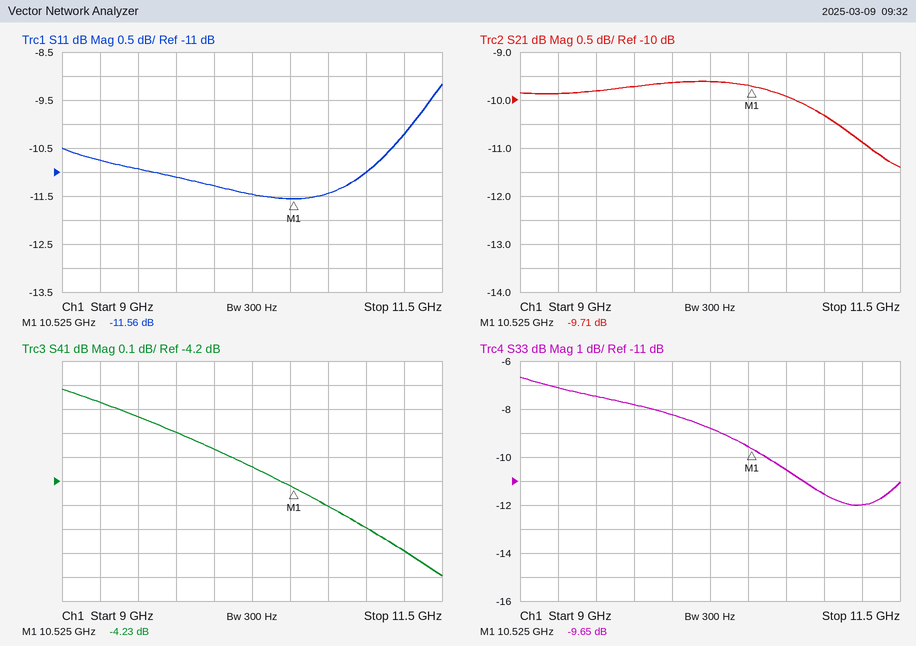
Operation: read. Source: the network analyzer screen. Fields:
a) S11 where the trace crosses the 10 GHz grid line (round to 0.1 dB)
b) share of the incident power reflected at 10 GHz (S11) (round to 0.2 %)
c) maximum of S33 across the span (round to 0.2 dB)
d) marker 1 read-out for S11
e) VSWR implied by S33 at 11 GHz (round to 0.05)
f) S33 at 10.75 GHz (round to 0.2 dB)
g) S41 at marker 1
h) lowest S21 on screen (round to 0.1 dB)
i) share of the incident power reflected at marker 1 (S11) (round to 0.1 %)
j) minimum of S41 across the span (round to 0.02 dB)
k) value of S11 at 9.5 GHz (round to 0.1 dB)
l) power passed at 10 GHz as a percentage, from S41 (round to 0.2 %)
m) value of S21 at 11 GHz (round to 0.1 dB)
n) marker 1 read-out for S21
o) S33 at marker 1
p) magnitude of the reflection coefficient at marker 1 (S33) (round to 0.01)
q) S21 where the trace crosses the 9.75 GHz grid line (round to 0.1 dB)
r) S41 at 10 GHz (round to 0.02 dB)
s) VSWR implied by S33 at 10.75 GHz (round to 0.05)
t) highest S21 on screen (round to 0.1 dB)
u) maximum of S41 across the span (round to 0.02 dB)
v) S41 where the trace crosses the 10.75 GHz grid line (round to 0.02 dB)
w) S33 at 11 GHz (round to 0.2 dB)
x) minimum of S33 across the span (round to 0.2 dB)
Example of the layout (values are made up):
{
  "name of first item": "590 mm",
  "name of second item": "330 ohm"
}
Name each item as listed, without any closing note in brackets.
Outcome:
{
  "S11 where the trace crosses the 10 GHz grid line": "-11.3 dB",
  "share of the incident power reflected at 10 GHz (S11)": "7.4 %",
  "maximum of S33 across the span": "-6.6 dB",
  "marker 1 read-out for S11": "-11.56 dB",
  "VSWR implied by S33 at 11 GHz": "1.70",
  "S33 at 10.75 GHz": "-10.6 dB",
  "S41 at marker 1": "-4.23 dB",
  "lowest S21 on screen": "-11.4 dB",
  "share of the incident power reflected at marker 1 (S11)": "7.0 %",
  "minimum of S41 across the span": "-4.60 dB",
  "value of S11 at 9.5 GHz": "-10.9 dB",
  "power passed at 10 GHz as a percentage, from S41": "39.2 %",
  "value of S21 at 11 GHz": "-10.3 dB",
  "marker 1 read-out for S21": "-9.71 dB",
  "S33 at marker 1": "-9.65 dB",
  "magnitude of the reflection coefficient at marker 1 (S33)": "0.33",
  "S21 where the trace crosses the 9.75 GHz grid line": "-9.7 dB",
  "S41 at 10 GHz": "-4.06 dB",
  "VSWR implied by S33 at 10.75 GHz": "1.85",
  "highest S21 on screen": "-9.6 dB",
  "maximum of S41 across the span": "-3.82 dB",
  "S41 where the trace crosses the 10.75 GHz grid line": "-4.30 dB",
  "S33 at 11 GHz": "-11.6 dB",
  "minimum of S33 across the span": "-12.0 dB"
}
